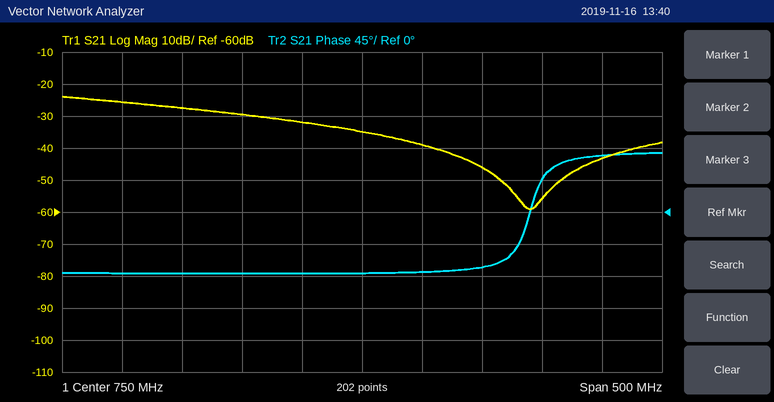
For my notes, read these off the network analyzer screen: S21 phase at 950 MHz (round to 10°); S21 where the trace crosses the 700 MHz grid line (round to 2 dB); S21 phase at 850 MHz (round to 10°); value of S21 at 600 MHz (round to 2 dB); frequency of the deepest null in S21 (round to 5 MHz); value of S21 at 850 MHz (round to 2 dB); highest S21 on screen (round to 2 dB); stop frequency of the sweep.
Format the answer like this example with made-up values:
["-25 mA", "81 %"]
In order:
["80°", "-32 dB", "-80°", "-28 dB", "890 MHz", "-46 dB", "-24 dB", "1 GHz"]
